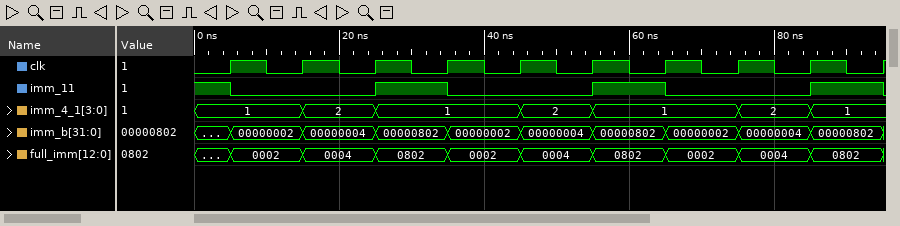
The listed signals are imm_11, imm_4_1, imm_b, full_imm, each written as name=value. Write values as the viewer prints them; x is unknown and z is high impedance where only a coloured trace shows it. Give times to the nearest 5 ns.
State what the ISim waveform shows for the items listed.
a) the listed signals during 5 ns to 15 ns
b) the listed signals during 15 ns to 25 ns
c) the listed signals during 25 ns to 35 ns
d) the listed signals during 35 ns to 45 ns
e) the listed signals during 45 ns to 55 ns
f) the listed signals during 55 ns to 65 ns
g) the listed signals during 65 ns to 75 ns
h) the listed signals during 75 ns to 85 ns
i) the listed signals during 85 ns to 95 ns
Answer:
imm_11=0, imm_4_1=1, imm_b=00000002, full_imm=0002
imm_11=0, imm_4_1=2, imm_b=00000004, full_imm=0004
imm_11=1, imm_4_1=1, imm_b=00000802, full_imm=0802
imm_11=0, imm_4_1=1, imm_b=00000002, full_imm=0002
imm_11=0, imm_4_1=2, imm_b=00000004, full_imm=0004
imm_11=1, imm_4_1=1, imm_b=00000802, full_imm=0802
imm_11=0, imm_4_1=1, imm_b=00000002, full_imm=0002
imm_11=0, imm_4_1=2, imm_b=00000004, full_imm=0004
imm_11=1, imm_4_1=1, imm_b=00000802, full_imm=0802
